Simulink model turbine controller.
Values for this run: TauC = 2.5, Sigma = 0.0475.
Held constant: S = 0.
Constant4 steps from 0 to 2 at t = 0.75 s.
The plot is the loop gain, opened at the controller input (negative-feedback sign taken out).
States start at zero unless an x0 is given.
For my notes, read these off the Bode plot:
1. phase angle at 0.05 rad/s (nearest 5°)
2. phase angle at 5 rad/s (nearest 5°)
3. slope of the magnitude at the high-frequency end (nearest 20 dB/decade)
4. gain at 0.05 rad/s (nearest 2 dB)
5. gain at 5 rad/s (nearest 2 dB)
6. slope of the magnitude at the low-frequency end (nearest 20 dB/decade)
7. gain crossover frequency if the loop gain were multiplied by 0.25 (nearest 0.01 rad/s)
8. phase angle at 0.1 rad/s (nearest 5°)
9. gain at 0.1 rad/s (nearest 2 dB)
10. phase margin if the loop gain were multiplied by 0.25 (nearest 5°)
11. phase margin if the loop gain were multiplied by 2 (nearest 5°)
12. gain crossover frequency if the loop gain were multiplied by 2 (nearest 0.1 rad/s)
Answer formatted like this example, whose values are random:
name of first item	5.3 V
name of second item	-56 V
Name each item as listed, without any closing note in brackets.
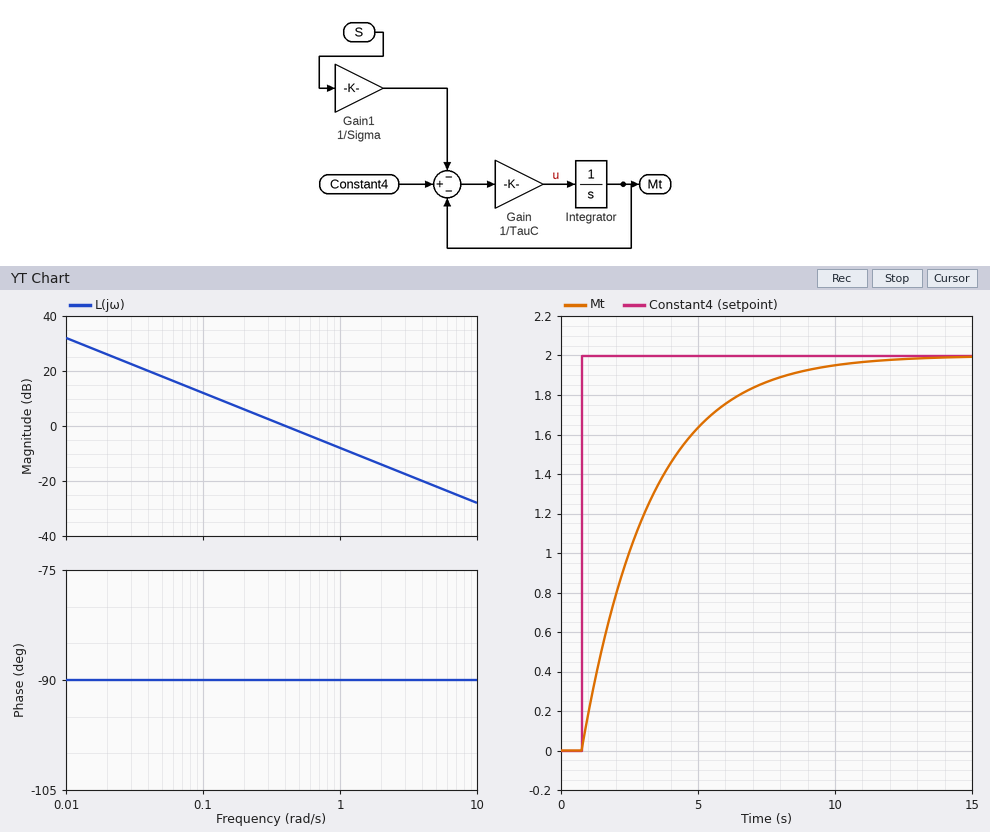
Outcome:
phase angle at 0.05 rad/s	-90°
phase angle at 5 rad/s	-90°
slope of the magnitude at the high-frequency end	-20 dB/decade
gain at 0.05 rad/s	18 dB
gain at 5 rad/s	-22 dB
slope of the magnitude at the low-frequency end	-20 dB/decade
gain crossover frequency if the loop gain were multiplied by 0.25	0.10 rad/s
phase angle at 0.1 rad/s	-90°
gain at 0.1 rad/s	12 dB
phase margin if the loop gain were multiplied by 0.25	90°
phase margin if the loop gain were multiplied by 2	90°
gain crossover frequency if the loop gain were multiplied by 2	0.8 rad/s
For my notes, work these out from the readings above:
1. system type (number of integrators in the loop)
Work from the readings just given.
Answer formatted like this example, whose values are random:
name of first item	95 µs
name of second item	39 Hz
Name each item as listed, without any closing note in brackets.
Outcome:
system type	1
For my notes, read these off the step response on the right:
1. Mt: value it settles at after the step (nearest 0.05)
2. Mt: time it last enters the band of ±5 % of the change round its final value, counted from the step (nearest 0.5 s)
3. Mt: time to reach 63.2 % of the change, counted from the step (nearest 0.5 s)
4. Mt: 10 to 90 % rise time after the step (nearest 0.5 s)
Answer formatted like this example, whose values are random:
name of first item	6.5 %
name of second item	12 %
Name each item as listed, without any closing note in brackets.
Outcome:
Mt: value it settles at after the step	2.00
Mt: time it last enters the band of ±5 % of the change round its final value, counted from the step	7.5 s
Mt: time to reach 63.2 % of the change, counted from the step	2.5 s
Mt: 10 to 90 % rise time after the step	5.5 s
